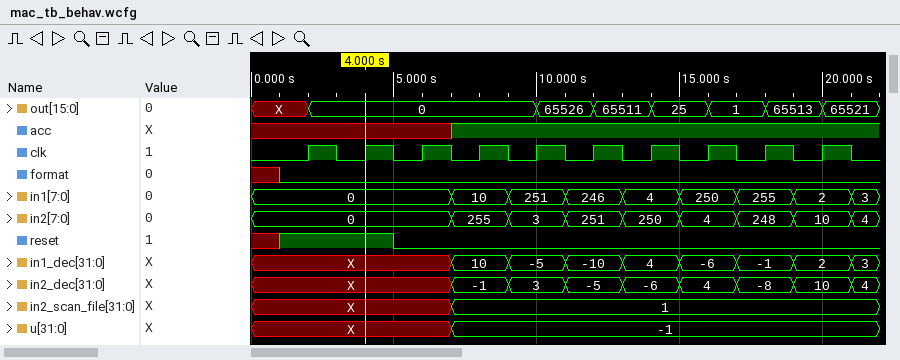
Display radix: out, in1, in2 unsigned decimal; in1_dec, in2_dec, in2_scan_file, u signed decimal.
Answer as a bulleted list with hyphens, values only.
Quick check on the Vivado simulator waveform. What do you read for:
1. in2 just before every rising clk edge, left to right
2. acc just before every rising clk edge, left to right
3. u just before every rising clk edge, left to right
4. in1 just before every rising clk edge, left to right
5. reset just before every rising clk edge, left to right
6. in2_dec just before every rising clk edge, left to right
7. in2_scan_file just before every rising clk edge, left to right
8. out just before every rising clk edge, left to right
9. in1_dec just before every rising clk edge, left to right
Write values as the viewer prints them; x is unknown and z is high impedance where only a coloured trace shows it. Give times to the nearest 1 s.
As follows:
- 0, 0, 0, 255, 3, 251, 250, 4, 248, 10
- x x x 1 1 1 1 1 1 1
- X, X, X, -1, -1, -1, -1, -1, -1, -1
- 0, 0, 0, 10, 251, 246, 4, 250, 255, 2
- 1 1 0 0 0 0 0 0 0 0
- X, X, X, -1, 3, -5, -6, 4, -8, 10
- X, X, X, 1, 1, 1, 1, 1, 1, 1
- X, 0, 0, 0, 0, 65526, 65511, 25, 1, 65513
- X, X, X, 10, -5, -10, 4, -6, -1, 2
